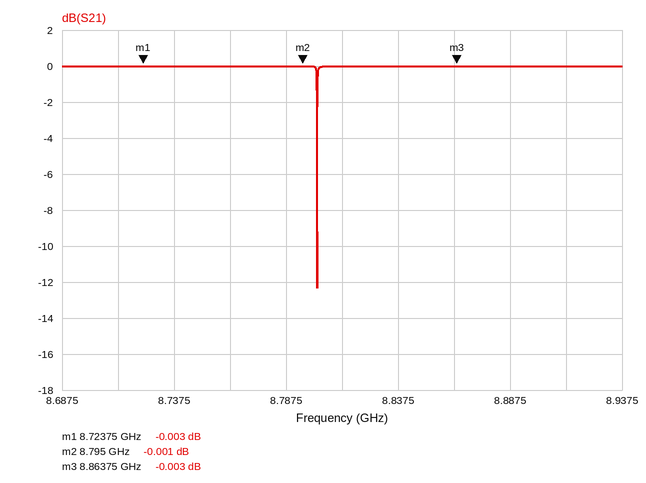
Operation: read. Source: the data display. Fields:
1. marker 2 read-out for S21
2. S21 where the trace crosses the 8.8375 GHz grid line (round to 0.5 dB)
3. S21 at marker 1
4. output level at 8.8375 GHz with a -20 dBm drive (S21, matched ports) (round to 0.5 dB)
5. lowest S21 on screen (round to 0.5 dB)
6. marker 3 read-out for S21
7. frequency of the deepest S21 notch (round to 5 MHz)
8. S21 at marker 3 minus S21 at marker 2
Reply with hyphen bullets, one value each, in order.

- -0.001 dB
- 0.0 dB
- -0.003 dB
- -20.0 dBm
- -12.5 dB
- -0.003 dB
- 8.800 GHz
- -0.002 dB
